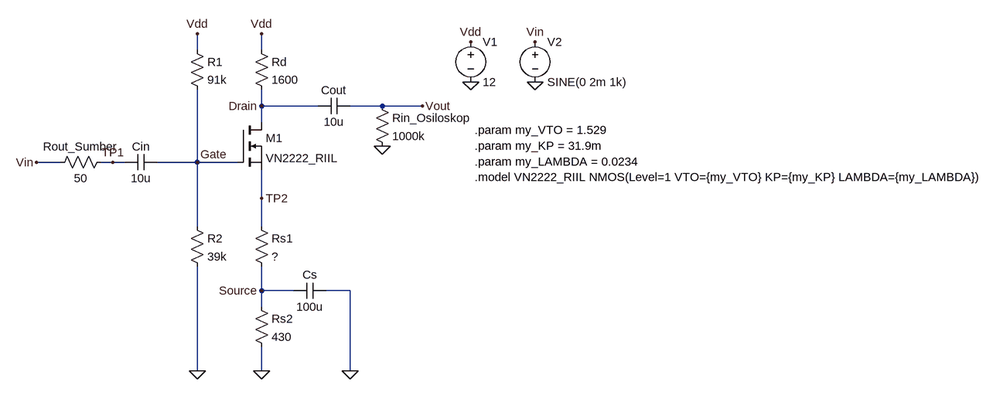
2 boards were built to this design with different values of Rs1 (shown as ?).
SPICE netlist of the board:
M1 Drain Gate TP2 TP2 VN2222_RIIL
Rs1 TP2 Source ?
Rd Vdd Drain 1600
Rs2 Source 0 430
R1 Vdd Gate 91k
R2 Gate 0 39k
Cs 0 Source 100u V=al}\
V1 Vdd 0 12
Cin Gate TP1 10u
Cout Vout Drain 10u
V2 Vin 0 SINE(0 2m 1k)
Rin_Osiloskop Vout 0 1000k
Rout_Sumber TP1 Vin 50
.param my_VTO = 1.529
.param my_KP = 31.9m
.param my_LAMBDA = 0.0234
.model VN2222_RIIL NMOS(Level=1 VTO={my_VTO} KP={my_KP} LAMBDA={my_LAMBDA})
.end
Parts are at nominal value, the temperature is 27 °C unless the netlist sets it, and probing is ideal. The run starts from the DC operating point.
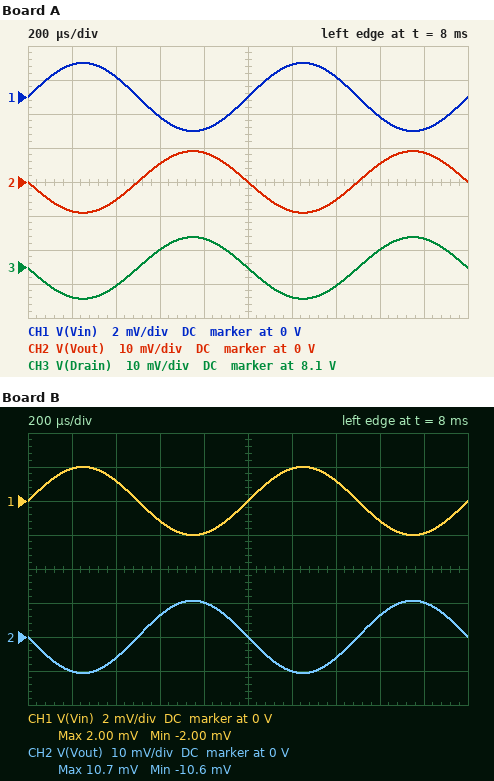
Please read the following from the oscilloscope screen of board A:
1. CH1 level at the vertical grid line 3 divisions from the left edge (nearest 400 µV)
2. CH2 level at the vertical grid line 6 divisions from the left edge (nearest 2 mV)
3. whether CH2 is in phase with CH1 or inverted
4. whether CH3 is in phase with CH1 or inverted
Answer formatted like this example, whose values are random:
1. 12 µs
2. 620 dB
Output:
1. -1.2 mV
2. -8 mV
3. inverted
4. inverted
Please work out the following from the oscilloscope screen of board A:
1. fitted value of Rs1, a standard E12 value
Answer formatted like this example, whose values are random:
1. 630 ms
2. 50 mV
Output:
1. 270 Ω
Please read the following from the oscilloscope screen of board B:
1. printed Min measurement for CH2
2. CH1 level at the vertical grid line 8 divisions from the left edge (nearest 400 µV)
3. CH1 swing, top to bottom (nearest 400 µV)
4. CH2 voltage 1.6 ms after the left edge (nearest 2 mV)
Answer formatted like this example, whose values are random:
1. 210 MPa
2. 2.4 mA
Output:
1. -10.6 mV
2. -1.2 mV
3. 4.0 mV
4. 6 mV
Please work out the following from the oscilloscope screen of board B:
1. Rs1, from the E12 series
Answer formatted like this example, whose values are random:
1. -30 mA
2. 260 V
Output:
1. 220 Ω
